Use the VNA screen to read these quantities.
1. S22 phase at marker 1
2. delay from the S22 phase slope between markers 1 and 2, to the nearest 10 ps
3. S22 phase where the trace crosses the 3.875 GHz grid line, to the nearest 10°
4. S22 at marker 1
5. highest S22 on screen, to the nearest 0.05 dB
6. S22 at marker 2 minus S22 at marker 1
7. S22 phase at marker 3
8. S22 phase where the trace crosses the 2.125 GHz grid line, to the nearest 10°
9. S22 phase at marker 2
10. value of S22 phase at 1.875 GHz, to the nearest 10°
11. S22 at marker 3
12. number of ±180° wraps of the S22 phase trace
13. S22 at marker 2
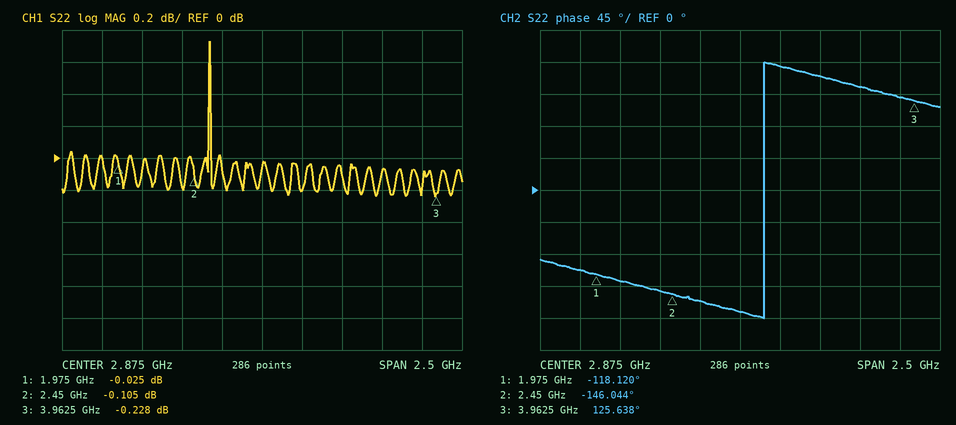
-118.120°
160 ps
130°
-0.025 dB
0.75 dB
-0.080 dB
125.638°
-130°
-146.044°
-110°
-0.228 dB
1
-0.105 dB
